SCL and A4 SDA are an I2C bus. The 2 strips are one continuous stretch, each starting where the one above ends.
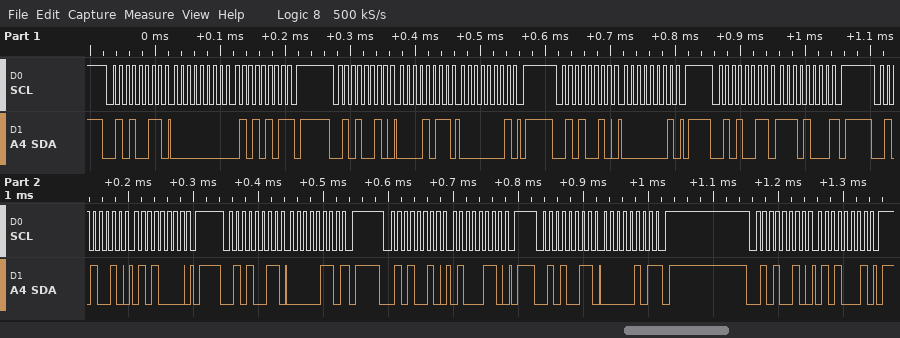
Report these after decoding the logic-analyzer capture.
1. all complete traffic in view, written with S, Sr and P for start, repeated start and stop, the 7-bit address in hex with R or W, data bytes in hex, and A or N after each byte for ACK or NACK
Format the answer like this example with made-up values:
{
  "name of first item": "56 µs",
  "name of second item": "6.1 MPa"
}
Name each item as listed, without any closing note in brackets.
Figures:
{
  "all complete traffic in view, written with S, Sr and P for start, repeated start and stop, the 7-bit address in hex with R or W, data bytes in hex, and A or N after each byte for ACK or NACK": "S 29R A 00 A 55 N P S 29W A 0B A 01 A P S 29W A 01 A P S 29R A E8 N P S 29W A 50 A P S 29R A 06 N P S 29W A 46 A P S 29R A 05 N P S 29W A 51 A P"
}
